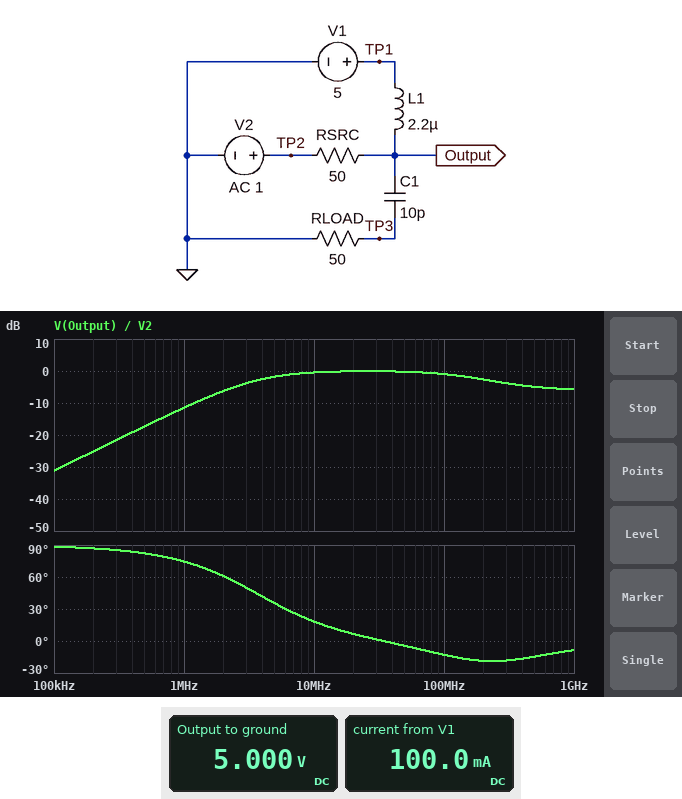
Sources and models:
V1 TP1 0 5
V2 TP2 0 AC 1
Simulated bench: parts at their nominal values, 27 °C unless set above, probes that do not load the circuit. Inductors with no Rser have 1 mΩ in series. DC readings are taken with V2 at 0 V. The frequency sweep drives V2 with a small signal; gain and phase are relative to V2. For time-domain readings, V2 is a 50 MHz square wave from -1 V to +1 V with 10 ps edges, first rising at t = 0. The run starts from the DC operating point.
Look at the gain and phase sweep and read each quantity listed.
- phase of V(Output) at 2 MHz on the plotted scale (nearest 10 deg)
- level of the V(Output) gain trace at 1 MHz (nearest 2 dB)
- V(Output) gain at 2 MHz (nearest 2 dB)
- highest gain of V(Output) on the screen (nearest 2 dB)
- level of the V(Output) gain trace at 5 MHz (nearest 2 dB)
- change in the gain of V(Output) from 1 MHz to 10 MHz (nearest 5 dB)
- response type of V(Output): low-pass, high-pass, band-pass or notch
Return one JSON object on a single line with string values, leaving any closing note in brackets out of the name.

{"phase of V(Output) at 2 MHz on the plotted scale": "60 deg", "level of the V(Output) gain trace at 1 MHz": "-12 dB", "V(Output) gain at 2 MHz": "-6 dB", "highest gain of V(Output) on the screen": "0 dB", "level of the V(Output) gain trace at 5 MHz": "-2 dB", "change in the gain of V(Output) from 1 MHz to 10 MHz": "10 dB", "response type of V(Output): low-pass, high-pass, band-pass or notch": "high-pass"}
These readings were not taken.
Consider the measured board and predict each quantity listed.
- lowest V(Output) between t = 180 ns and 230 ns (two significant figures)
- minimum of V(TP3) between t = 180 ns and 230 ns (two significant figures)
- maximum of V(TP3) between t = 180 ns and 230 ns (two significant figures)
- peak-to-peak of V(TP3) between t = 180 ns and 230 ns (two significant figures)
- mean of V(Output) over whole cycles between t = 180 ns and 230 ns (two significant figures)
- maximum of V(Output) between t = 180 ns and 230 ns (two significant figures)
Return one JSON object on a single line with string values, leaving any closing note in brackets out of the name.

{"lowest V(Output) between t = 180 ns and 230 ns": "4.0 V", "minimum of V(TP3) between t = 180 ns and 230 ns": "-1.0 V", "maximum of V(TP3) between t = 180 ns and 230 ns": "1.0 V", "peak-to-peak of V(TP3) between t = 180 ns and 230 ns": "2.0 V", "mean of V(Output) over whole cycles between t = 180 ns and 230 ns": "5.0 V", "maximum of V(Output) between t = 180 ns and 230 ns": "6.0 V"}
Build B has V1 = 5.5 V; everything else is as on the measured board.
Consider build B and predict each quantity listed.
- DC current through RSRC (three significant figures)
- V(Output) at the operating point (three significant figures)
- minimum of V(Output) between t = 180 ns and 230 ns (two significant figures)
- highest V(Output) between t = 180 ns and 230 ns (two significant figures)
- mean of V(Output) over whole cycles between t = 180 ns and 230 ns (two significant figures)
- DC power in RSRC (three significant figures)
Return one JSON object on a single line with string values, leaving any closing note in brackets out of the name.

{"DC current through RSRC": "110 mA", "V(Output) at the operating point": "5.50 V", "minimum of V(Output) between t = 180 ns and 230 ns": "4.5 V", "highest V(Output) between t = 180 ns and 230 ns": "6.5 V", "mean of V(Output) over whole cycles between t = 180 ns and 230 ns": "5.5 V", "DC power in RSRC": "605 mW"}
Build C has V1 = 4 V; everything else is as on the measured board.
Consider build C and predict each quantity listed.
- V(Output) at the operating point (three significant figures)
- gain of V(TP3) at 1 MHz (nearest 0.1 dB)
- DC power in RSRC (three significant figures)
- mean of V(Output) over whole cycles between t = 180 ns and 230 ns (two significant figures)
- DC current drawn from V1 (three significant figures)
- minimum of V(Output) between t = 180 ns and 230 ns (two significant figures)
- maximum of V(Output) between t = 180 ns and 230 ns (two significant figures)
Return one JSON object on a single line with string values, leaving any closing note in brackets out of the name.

{"V(Output) at the operating point": "4.00 V", "gain of V(TP3) at 1 MHz": "-61.5 dB", "DC power in RSRC": "320 mW", "mean of V(Output) over whole cycles between t = 180 ns and 230 ns": "4.0 V", "DC current drawn from V1": "80.0 mA", "minimum of V(Output) between t = 180 ns and 230 ns": "3.0 V", "maximum of V(Output) between t = 180 ns and 230 ns": "5.0 V"}
